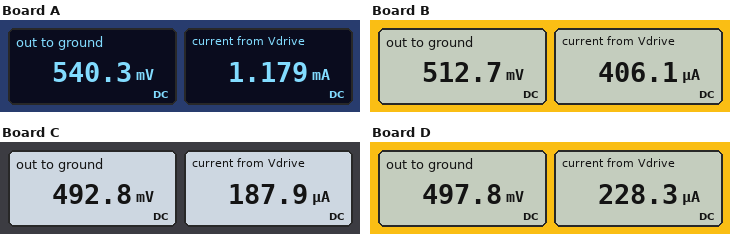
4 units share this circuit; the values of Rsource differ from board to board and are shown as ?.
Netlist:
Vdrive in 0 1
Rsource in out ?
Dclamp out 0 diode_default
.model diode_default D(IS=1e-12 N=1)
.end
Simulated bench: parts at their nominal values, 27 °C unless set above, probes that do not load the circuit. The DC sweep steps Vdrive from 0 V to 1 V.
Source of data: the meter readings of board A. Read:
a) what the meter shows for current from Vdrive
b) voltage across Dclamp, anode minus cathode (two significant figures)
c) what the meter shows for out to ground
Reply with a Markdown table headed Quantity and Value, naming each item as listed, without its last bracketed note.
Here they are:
| Quantity | Value |
|---|---|
| what the meter shows for current from Vdrive | 1.179 mA |
| voltage across Dclamp, anode minus cathode | 540 mV |
| what the meter shows for out to ground | 540.3 mV |
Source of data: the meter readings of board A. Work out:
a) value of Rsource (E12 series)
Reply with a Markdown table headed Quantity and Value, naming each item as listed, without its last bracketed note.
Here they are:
| Quantity | Value |
|---|---|
| value of Rsource | 390 Ω |
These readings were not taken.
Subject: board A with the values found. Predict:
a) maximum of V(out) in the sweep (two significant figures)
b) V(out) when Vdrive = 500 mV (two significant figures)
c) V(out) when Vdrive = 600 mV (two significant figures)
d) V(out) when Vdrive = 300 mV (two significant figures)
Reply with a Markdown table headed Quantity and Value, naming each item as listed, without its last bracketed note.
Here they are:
| Quantity | Value |
|---|---|
| maximum of V(out) in the sweep | 540 mV |
| V(out) when Vdrive = 500 mV | 470 mV |
| V(out) when Vdrive = 600 mV | 500 mV |
| V(out) when Vdrive = 300 mV | 300 mV |
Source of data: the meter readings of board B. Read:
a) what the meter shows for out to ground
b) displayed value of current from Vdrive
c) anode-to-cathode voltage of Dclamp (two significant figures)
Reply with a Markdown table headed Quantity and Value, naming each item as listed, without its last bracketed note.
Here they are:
| Quantity | Value |
|---|---|
| what the meter shows for out to ground | 512.7 mV |
| displayed value of current from Vdrive | 406.1 µA |
| anode-to-cathode voltage of Dclamp | 510 mV |
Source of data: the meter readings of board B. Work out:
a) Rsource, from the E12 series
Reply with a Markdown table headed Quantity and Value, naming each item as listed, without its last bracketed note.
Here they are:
| Quantity | Value |
|---|---|
| Rsource, from the E12 series | 1.2 kΩ |
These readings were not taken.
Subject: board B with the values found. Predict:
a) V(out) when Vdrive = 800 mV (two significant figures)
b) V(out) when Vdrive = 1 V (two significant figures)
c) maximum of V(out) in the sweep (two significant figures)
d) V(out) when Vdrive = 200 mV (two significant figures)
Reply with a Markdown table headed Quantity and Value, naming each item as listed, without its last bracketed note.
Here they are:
| Quantity | Value |
|---|---|
| V(out) when Vdrive = 800 mV | 500 mV |
| V(out) when Vdrive = 1 V | 510 mV |
| maximum of V(out) in the sweep | 510 mV |
| V(out) when Vdrive = 200 mV | 200 mV |
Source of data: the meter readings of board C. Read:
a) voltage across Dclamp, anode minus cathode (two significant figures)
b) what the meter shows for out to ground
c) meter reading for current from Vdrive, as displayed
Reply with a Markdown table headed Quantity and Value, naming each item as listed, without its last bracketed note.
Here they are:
| Quantity | Value |
|---|---|
| voltage across Dclamp, anode minus cathode | 490 mV |
| what the meter shows for out to ground | 492.8 mV |
| meter reading for current from Vdrive, as displayed | 187.9 µA |
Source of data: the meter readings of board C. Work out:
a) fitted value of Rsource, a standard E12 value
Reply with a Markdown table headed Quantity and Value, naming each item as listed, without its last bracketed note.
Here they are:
| Quantity | Value |
|---|---|
| fitted value of Rsource, a standard E12 value | 2.7 kΩ |
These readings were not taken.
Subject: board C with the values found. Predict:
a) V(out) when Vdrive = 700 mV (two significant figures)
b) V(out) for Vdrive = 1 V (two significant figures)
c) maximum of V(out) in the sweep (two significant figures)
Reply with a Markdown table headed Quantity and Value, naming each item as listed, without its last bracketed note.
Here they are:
| Quantity | Value |
|---|---|
| V(out) when Vdrive = 700 mV | 470 mV |
| V(out) for Vdrive = 1 V | 490 mV |
| maximum of V(out) in the sweep | 490 mV |
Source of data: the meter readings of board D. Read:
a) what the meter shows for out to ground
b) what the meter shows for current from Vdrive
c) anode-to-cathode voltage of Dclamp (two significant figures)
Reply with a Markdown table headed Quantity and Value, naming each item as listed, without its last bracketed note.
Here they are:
| Quantity | Value |
|---|---|
| what the meter shows for out to ground | 497.8 mV |
| what the meter shows for current from Vdrive | 228.3 µA |
| anode-to-cathode voltage of Dclamp | 500 mV |
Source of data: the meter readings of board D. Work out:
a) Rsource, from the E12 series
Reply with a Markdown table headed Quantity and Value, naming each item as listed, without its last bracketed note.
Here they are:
| Quantity | Value |
|---|---|
| Rsource, from the E12 series | 2.2 kΩ |
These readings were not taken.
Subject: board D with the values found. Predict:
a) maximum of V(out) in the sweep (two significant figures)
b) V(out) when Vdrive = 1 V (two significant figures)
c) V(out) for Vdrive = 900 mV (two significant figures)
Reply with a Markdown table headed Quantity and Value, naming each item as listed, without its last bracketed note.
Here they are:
| Quantity | Value |
|---|---|
| maximum of V(out) in the sweep | 500 mV |
| V(out) when Vdrive = 1 V | 500 mV |
| V(out) for Vdrive = 900 mV | 490 mV |
